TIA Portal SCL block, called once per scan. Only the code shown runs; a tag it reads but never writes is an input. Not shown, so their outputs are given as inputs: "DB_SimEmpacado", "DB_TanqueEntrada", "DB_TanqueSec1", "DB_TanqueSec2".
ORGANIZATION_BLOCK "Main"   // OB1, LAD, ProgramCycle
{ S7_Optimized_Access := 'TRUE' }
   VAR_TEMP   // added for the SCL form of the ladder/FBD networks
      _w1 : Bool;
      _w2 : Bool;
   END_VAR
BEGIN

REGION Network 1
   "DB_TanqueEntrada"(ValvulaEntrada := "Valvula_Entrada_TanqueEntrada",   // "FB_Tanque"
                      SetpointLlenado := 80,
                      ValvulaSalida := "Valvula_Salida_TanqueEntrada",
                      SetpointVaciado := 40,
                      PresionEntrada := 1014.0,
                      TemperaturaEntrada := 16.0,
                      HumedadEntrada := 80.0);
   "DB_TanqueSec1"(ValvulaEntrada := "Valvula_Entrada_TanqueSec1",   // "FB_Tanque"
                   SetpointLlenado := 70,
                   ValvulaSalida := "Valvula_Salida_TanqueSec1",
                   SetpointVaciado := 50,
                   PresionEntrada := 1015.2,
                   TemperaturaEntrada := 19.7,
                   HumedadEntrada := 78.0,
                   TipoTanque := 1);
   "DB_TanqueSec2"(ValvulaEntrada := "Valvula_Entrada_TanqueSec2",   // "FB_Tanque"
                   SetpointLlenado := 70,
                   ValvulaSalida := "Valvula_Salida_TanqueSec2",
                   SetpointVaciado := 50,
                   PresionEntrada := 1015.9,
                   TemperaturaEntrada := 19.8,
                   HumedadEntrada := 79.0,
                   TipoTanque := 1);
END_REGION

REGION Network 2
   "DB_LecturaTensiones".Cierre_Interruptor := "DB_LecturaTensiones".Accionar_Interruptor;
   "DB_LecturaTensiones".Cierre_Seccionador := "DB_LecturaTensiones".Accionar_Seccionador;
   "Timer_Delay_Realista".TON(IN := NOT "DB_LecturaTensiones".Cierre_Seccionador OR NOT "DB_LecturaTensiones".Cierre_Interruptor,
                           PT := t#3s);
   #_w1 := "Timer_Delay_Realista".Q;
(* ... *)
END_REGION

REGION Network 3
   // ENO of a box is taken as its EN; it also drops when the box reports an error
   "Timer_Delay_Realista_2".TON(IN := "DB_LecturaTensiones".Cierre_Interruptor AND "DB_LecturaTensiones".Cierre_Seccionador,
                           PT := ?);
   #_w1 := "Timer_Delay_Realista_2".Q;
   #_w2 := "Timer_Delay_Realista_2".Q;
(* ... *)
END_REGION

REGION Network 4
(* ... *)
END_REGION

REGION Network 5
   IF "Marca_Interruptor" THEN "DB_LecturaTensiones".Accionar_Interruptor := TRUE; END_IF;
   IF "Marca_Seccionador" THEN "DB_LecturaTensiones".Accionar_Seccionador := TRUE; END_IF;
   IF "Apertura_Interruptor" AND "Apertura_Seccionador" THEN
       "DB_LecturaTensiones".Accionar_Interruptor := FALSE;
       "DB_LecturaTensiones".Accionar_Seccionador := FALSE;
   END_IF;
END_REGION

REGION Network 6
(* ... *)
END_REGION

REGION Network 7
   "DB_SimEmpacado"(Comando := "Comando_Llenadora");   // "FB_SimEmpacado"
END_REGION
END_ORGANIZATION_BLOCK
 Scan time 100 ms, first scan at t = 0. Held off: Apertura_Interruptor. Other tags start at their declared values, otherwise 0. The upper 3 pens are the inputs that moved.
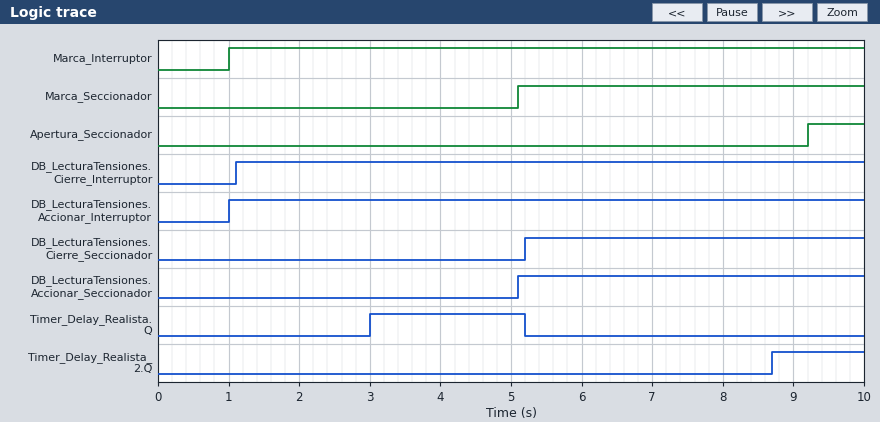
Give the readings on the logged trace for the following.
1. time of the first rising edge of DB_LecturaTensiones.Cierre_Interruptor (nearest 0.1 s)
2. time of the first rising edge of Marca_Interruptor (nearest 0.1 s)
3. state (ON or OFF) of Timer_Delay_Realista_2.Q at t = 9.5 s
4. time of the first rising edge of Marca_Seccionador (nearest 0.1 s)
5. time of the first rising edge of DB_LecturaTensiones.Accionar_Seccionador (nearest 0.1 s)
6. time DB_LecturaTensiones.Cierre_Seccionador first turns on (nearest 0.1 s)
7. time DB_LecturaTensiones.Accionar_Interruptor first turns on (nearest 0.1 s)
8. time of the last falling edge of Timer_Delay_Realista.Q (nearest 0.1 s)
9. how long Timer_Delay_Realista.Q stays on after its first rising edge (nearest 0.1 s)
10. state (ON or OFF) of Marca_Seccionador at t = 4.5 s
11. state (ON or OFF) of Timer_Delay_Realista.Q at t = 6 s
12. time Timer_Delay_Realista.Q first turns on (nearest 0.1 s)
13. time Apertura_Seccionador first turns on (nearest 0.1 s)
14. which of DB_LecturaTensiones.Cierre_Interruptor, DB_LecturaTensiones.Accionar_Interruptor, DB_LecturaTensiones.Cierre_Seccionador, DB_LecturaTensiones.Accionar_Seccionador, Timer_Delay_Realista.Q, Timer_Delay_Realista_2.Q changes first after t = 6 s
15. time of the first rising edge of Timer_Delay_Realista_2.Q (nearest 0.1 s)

1.1 s
1.0 s
ON
5.1 s
5.1 s
5.2 s
1.0 s
5.2 s
2.2 s
OFF
OFF
3.0 s
9.2 s
Timer_Delay_Realista_2.Q
8.7 s
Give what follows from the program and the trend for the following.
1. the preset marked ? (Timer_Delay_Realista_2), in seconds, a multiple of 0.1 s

3.5 s
